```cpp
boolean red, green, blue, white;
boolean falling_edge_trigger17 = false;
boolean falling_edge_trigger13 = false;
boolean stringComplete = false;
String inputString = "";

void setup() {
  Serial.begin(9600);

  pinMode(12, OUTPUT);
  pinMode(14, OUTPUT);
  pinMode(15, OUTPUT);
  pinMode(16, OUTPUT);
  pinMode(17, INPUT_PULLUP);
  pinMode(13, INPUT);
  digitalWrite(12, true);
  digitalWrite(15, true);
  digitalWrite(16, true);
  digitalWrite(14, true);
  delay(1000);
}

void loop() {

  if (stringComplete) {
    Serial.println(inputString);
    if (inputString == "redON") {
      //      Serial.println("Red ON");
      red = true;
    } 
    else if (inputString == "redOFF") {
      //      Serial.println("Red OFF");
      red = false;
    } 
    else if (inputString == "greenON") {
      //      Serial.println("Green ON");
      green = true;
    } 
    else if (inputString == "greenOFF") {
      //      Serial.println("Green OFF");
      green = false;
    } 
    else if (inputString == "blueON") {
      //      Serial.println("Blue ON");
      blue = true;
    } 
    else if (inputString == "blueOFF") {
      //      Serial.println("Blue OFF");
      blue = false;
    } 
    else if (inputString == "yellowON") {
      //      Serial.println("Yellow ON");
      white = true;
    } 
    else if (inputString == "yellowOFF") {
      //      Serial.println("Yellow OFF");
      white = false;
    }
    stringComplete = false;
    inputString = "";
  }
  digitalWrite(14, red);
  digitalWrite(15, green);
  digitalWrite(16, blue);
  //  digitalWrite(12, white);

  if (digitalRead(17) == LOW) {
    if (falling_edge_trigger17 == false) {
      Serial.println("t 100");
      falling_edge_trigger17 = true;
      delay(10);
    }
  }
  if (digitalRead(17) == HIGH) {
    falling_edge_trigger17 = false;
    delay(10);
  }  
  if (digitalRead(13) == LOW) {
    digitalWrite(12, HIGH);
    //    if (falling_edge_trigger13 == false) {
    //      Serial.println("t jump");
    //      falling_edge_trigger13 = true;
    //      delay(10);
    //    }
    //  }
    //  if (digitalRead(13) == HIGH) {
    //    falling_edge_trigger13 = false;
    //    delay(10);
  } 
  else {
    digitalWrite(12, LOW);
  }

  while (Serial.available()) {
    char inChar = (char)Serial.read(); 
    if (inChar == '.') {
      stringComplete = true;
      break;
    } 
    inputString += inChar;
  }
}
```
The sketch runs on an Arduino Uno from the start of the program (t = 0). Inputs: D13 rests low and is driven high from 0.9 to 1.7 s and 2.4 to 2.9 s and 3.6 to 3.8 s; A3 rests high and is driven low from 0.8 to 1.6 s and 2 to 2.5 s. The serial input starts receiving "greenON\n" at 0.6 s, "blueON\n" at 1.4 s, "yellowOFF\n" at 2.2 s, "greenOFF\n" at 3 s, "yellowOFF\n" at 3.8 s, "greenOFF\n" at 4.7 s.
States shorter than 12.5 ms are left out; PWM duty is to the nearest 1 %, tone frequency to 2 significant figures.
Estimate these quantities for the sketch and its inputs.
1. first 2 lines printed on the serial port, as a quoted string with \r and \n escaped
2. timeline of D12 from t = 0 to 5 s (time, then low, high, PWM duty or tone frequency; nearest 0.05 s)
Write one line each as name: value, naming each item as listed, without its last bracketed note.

first 2 lines printed on the serial port, as a quoted string with \r and \n escaped: "t 100\r\nt 100\r\n"
timeline of D12 from t = 0 to 5 s: 0 s high; 1 s low; 1.7 s high; 2.4 s low; 2.9 s high; 3.6 s low; 3.8 s high
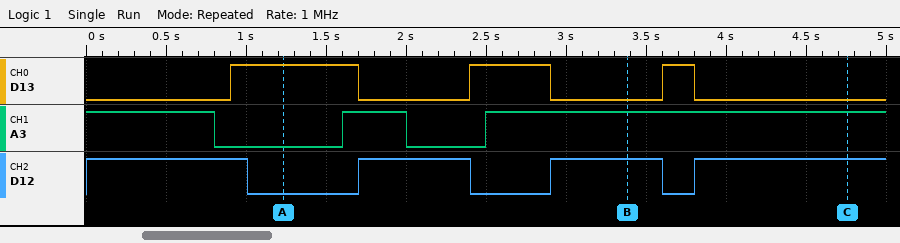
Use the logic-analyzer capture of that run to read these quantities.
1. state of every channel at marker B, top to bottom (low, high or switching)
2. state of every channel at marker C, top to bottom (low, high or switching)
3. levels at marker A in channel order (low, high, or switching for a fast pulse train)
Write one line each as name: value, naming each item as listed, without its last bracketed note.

state of every channel at marker B, top to bottom: D13 low, A3 high, D12 high
state of every channel at marker C, top to bottom: D13 low, A3 high, D12 high
levels at marker A in channel order: D13 high, A3 low, D12 low
